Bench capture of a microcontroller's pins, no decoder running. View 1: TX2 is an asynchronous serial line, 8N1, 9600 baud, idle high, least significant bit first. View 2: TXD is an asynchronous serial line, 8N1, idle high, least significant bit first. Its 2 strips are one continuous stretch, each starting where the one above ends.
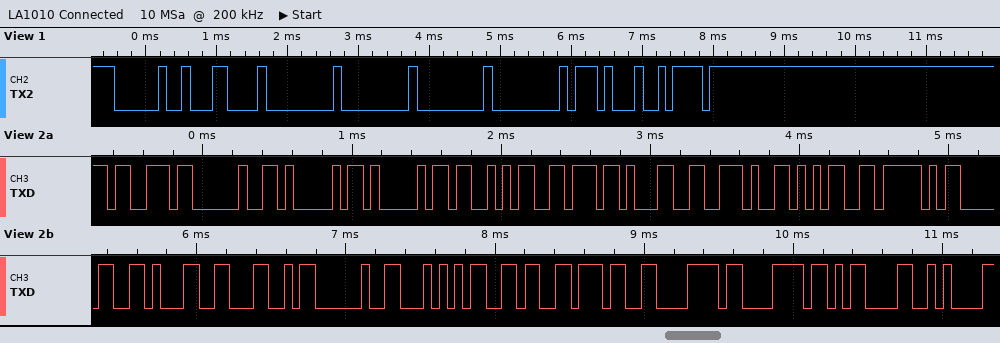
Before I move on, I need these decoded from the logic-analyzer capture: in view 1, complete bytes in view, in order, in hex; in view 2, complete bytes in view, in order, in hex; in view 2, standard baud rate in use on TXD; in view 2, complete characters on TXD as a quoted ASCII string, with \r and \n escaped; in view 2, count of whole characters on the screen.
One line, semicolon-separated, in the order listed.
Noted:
20 0C 00 00 00 00 17 7A; 73 20 41 41 53 76 31 2E 35 5F 30 31 4C 20 54 36 37 78 78 0D 0A; 19200 baud; "s AASv1.5_01L T67xx\r\n"; 21
